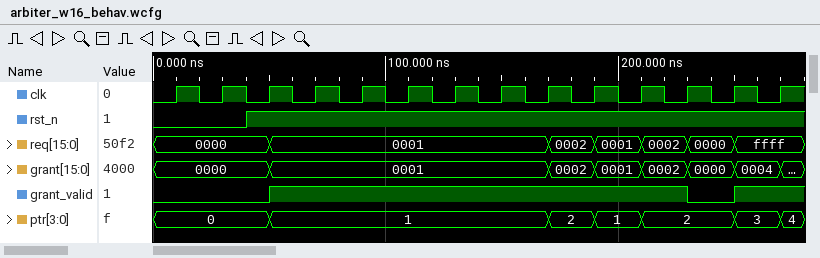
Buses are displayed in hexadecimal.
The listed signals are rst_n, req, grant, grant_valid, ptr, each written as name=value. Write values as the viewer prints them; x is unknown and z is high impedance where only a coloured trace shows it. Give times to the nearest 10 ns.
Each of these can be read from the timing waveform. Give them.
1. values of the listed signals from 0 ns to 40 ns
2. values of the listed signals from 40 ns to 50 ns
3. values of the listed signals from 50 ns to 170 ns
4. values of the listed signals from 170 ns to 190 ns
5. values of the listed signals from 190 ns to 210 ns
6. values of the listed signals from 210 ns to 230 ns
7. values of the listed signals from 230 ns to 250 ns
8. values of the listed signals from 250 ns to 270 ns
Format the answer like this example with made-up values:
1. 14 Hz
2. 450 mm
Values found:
1. rst_n=0, req=0000, grant=0000, grant_valid=0, ptr=0
2. rst_n=1, req=0000, grant=0000, grant_valid=0, ptr=0
3. rst_n=1, req=0001, grant=0001, grant_valid=1, ptr=1
4. rst_n=1, req=0002, grant=0002, grant_valid=1, ptr=2
5. rst_n=1, req=0001, grant=0001, grant_valid=1, ptr=1
6. rst_n=1, req=0002, grant=0002, grant_valid=1, ptr=2
7. rst_n=1, req=0000, grant=0000, grant_valid=0, ptr=2
8. rst_n=1, req=ffff, grant=0004, grant_valid=1, ptr=3
